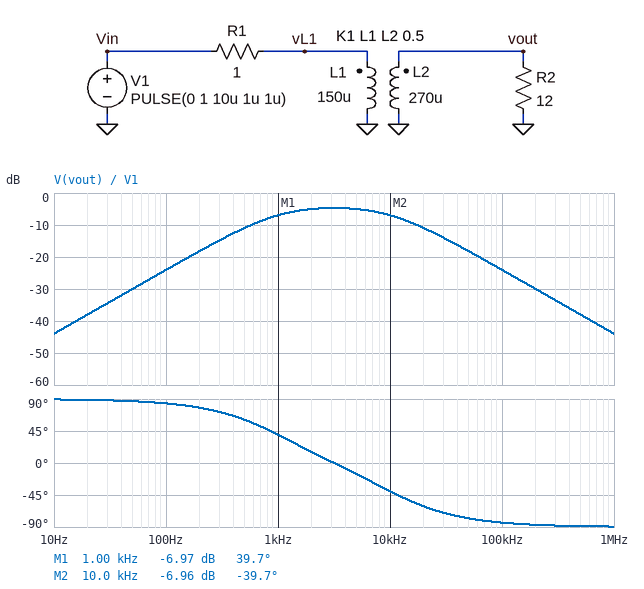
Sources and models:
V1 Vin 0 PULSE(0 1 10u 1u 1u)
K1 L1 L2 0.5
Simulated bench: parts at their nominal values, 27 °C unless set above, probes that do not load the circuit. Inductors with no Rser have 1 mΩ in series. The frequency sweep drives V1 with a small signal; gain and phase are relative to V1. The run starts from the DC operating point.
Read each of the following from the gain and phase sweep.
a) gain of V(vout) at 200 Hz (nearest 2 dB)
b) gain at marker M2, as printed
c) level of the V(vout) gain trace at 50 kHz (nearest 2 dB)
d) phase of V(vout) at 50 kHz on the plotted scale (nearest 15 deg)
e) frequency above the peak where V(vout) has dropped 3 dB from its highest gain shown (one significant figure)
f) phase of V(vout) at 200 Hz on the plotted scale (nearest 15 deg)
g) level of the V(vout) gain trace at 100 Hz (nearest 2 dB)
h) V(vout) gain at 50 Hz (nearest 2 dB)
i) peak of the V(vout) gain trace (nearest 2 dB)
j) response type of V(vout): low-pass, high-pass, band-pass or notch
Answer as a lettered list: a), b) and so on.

a) -18 dB
b) -6.96 dB
c) -18 dB
d) -75 deg
e) 10 kHz
f) 75 deg
g) -24 dB
h) -30 dB
i) -4 dB
j) band-pass
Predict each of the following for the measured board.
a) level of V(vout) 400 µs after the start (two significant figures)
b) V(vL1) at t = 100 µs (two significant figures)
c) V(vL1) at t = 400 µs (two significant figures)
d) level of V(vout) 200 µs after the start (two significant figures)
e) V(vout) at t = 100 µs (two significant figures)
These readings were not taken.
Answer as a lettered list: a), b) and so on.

a) 59 mV
b) 540 mV
c) 80 mV
d) 210 mV
e) 400 mV
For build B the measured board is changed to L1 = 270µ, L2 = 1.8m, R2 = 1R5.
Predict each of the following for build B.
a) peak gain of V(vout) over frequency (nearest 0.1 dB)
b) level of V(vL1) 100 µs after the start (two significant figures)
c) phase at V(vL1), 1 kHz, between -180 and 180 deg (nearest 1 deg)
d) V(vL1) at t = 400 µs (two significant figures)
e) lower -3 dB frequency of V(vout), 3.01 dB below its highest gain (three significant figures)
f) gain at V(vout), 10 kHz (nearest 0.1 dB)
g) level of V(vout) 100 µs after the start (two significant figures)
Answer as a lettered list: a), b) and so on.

a) -12.5 dB
b) 650 mV
c) 37 deg
d) 170 mV
e) 98.3 Hz
f) -32.9 dB
g) 99 mV
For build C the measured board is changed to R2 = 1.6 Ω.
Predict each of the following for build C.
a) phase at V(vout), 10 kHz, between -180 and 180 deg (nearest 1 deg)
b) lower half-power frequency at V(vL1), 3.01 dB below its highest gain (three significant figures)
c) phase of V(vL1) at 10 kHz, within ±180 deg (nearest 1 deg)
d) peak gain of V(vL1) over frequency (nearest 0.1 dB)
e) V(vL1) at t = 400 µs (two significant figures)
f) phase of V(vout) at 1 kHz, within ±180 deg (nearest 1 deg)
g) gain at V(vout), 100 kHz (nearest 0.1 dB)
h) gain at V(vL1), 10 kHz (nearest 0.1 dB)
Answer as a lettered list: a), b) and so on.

a) -75 deg
b) 1.46 kHz
c) 8 deg
d) 0 dB
e) 92 mV
f) 7 deg
g) -41.5 dB
h) -0.1 dB
